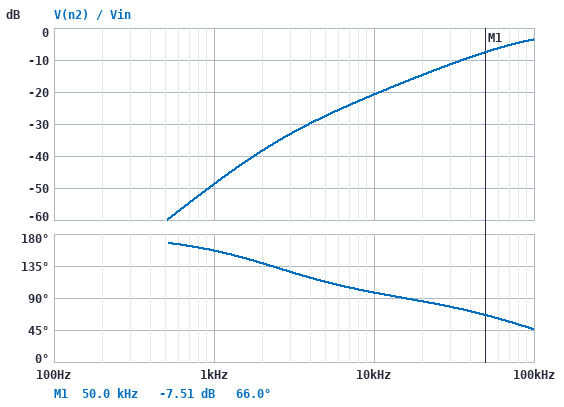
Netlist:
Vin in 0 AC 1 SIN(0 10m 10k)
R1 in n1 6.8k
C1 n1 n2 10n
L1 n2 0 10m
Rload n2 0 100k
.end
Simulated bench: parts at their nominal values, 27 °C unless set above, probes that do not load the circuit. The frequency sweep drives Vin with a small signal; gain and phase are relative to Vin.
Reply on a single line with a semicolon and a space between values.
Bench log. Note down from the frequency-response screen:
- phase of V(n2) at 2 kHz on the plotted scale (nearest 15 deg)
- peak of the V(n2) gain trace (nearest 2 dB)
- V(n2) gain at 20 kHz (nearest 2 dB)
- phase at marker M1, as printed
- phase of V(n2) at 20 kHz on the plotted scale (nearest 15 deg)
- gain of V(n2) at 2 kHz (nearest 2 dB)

135 deg; -4 dB; -14 dB; 66.0 deg; 90 deg; -38 dB
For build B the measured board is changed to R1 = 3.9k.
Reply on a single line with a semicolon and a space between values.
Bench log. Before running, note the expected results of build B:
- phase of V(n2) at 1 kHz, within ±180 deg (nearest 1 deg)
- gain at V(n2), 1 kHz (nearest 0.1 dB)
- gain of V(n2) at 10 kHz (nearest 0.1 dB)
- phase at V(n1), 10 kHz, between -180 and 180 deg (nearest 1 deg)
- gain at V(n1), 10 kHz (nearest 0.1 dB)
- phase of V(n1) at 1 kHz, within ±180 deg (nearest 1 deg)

166 deg; -48.3 dB; -16.1 dB; -76 deg; -12.4 dB; -14 deg
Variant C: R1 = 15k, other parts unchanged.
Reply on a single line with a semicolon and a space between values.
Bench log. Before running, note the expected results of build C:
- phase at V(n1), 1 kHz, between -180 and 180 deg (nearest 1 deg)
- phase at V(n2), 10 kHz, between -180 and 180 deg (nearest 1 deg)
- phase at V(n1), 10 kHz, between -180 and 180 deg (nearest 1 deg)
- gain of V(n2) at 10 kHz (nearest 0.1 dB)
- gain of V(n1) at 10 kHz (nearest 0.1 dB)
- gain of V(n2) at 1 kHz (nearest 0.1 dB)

-43 deg; 93 deg; -86 deg; -27.6 dB; -23.9 dB; -50.8 dB
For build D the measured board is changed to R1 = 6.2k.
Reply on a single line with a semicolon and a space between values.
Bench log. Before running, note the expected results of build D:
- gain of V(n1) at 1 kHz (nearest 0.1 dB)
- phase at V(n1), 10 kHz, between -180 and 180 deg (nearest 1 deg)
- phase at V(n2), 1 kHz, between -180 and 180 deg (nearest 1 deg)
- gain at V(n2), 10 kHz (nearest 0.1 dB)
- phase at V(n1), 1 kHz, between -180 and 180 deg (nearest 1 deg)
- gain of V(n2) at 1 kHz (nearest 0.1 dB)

-0.6 dB; -81 deg; 159 deg; -20.0 dB; -21 deg; -48.7 dB
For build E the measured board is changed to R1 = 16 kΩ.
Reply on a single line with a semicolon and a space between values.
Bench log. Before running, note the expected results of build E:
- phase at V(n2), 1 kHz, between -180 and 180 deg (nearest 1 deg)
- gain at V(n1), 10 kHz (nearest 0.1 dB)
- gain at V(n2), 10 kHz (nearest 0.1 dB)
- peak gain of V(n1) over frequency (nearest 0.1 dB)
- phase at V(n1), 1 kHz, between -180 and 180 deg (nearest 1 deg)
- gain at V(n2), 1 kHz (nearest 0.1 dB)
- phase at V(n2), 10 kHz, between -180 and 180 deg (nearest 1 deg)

135 deg; -24.4 dB; -28.1 dB; 0 dB; -45 deg; -51.1 dB; 93 deg
